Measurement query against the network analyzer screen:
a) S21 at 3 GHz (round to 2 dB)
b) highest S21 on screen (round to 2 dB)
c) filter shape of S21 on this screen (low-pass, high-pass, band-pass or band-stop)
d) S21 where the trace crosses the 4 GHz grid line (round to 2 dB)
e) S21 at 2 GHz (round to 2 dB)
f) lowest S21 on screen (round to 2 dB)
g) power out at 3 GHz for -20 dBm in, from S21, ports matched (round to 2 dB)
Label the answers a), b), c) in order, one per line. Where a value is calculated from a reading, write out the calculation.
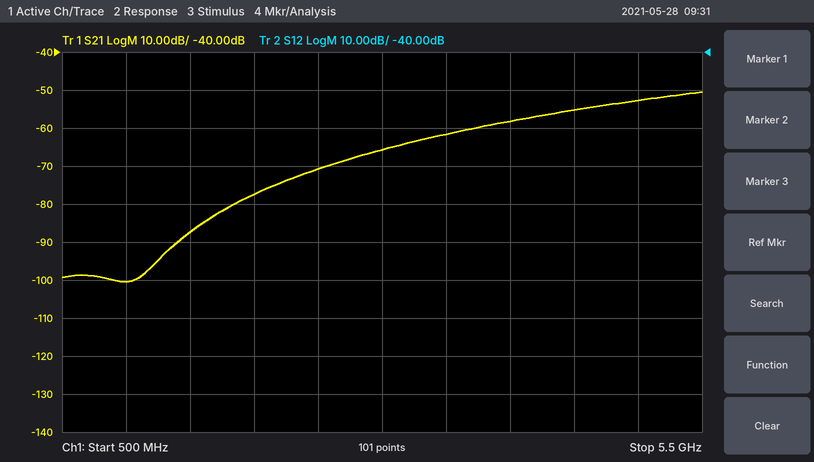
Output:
a) -66 dB
b) -50 dB
c) high-pass
d) -58 dB
e) -78 dB
f) -100 dB
g) -20 dBm + (-66 dB) = -86 dBm
